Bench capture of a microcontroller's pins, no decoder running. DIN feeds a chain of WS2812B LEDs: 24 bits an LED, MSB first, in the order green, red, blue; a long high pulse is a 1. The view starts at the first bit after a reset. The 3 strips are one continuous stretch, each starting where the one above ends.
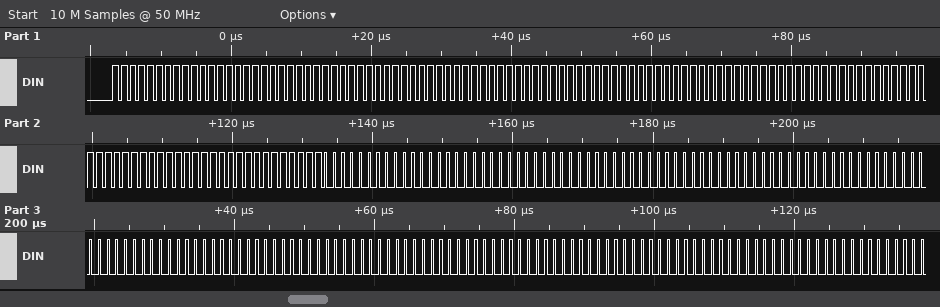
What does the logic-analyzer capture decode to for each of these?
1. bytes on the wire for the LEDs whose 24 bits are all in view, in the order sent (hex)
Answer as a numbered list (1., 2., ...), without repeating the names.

1. FF FF FF FF FF FF FF FF FF FF FF FF FF FF FF 00 00 00 00 00 00 00 00 00 00 00 00 00 00 00 00 00 00
